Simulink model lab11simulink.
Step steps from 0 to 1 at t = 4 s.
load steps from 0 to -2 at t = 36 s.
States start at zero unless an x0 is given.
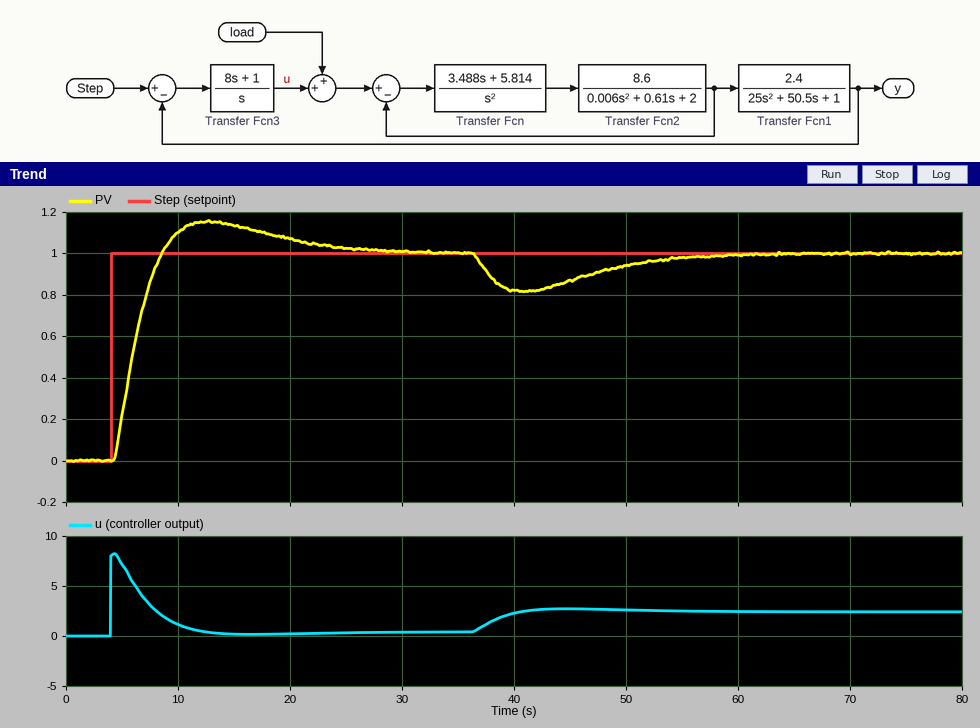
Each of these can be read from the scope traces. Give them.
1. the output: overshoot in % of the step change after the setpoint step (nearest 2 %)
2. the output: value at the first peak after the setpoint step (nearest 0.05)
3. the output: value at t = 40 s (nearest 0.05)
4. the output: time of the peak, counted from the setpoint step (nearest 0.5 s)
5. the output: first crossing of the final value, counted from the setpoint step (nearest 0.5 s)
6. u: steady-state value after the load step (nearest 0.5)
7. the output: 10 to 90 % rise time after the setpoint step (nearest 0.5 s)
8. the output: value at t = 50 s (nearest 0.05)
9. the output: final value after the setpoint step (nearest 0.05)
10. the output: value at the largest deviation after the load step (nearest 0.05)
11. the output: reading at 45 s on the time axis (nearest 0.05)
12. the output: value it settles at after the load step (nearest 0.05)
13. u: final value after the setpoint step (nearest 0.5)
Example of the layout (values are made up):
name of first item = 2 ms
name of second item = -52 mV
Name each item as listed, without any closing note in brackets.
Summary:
the output: overshoot in % of the step change after the setpoint step = 16 %
the output: value at the first peak after the setpoint step = 1.15
the output: value at t = 40 s = 0.80
the output: time of the peak, counted from the setpoint step = 8.5 s
the output: first crossing of the final value, counted from the setpoint step = 4.5 s
u: steady-state value after the load step = 2.5
the output: 10 to 90 % rise time after the setpoint step = 3.0 s
the output: value at t = 50 s = 0.95
the output: final value after the setpoint step = 1.00
the output: value at the largest deviation after the load step = 0.80
the output: reading at 45 s on the time axis = 0.85
the output: value it settles at after the load step = 1.00
u: final value after the setpoint step = 0.5
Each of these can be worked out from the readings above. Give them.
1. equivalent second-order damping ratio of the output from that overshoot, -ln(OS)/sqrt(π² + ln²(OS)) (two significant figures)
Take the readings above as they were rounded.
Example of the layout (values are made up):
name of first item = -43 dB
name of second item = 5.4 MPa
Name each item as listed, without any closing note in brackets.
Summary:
equivalent second-order damping ratio of the output from that overshoot, -ln(OS)/sqrt(π² + ln²(OS)) = 0.50
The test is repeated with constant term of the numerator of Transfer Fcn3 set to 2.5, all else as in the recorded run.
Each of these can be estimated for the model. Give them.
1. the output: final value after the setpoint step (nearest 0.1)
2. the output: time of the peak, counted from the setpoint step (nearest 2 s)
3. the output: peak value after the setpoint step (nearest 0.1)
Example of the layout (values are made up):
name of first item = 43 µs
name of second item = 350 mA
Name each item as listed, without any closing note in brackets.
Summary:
the output: final value after the setpoint step = 1.0
the output: time of the peak, counted from the setpoint step = 6 s
the output: peak value after the setpoint step = 1.3
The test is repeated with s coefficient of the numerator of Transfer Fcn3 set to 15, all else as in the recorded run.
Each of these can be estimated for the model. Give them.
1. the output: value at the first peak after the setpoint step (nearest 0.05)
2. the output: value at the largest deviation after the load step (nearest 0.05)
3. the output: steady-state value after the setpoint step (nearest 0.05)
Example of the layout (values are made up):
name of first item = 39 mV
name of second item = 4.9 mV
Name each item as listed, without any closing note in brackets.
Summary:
the output: value at the first peak after the setpoint step = 1.05
the output: value at the largest deviation after the load step = 0.90
the output: steady-state value after the setpoint step = 1.00
